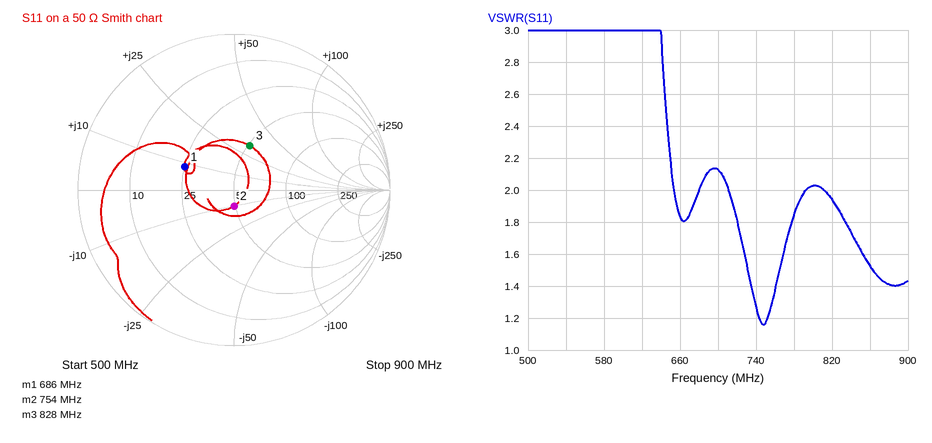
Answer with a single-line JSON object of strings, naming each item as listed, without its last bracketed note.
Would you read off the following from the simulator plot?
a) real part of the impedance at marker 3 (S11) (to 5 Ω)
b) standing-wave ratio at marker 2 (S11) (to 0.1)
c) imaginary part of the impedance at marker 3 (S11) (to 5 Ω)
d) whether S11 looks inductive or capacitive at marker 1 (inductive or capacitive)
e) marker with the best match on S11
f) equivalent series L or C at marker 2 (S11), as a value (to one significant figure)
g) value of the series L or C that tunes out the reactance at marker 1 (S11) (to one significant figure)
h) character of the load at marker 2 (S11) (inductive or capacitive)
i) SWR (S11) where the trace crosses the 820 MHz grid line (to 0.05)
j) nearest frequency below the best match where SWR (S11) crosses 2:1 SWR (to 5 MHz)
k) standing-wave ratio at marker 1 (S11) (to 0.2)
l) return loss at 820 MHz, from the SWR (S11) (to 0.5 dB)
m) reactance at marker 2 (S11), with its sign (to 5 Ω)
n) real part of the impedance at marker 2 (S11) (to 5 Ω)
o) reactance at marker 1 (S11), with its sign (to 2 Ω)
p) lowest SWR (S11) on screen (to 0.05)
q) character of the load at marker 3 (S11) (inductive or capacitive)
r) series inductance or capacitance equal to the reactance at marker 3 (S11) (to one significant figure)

{"real part of the impedance at marker 3 (S11)": "50 Ω", "standing-wave ratio at marker 2 (S11)": "1.2", "imaginary part of the impedance at marker 3 (S11)": "+30 Ω", "whether S11 looks inductive or capacitive at marker 1": "inductive", "marker with the best match on S11": "marker 2", "equivalent series L or C at marker 2 (S11), as a value": "20 pF", "value of the series L or C that tunes out the reactance at marker 1 (S11)": "30 pF", "character of the load at marker 2 (S11)": "capacitive", "SWR (S11) where the trace crosses the 820 MHz grid line": "1.95", "nearest frequency below the best match where SWR (S11) crosses 2:1 SWR": "710 MHz", "standing-wave ratio at marker 1 (S11)": "2.0", "return loss at 820 MHz, from the SWR (S11)": "10.0 dB", "reactance at marker 2 (S11), with its sign": "-10 Ω", "real part of the impedance at marker 2 (S11)": "50 Ω", "reactance at marker 1 (S11), with its sign": "+8 Ω", "lowest SWR (S11) on screen": "1.15", "character of the load at marker 3 (S11)": "inductive", "series inductance or capacitance equal to the reactance at marker 3 (S11)": "6 nH"}
